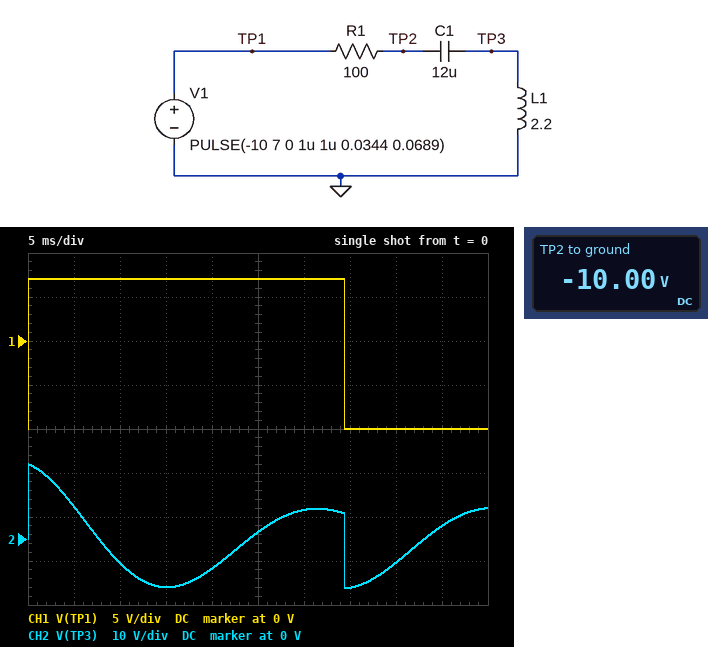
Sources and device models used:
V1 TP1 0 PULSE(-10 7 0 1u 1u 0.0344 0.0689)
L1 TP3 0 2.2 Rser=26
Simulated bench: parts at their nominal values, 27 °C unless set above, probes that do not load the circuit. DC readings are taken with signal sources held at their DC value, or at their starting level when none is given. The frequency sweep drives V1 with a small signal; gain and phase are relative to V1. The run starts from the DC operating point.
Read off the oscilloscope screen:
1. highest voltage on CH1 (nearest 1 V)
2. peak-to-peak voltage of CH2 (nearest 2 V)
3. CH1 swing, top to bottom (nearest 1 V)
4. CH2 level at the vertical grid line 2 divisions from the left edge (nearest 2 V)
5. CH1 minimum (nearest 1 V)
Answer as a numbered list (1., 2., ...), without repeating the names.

1. 7 V
2. 28 V
3. 17 V
4. -6 V
5. -10 V
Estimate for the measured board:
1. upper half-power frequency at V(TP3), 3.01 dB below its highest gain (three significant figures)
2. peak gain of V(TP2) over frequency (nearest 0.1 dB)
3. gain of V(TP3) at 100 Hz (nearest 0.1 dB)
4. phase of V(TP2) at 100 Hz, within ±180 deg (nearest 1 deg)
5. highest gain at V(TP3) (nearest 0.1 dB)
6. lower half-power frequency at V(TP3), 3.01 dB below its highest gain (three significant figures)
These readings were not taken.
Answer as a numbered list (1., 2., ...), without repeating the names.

1. 38.0 Hz
2. 0 dB
3. 0.8 dB
4. 5 deg
5. 10.7 dB
6. 27.7 Hz
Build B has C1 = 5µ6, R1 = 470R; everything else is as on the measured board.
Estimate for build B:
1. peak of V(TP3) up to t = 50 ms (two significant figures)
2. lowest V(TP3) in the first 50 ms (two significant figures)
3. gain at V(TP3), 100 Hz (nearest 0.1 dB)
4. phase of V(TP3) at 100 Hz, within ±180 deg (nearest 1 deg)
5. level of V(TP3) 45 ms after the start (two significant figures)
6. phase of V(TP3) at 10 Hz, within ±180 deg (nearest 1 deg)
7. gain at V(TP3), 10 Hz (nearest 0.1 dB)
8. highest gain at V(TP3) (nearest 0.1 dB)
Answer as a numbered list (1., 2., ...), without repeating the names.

1. 17 V
2. -17 V
3. 1.2 dB
4. 23 deg
5. 5.6 V
6. 159 deg
7. -25.8 dB
8. 2.8 dB
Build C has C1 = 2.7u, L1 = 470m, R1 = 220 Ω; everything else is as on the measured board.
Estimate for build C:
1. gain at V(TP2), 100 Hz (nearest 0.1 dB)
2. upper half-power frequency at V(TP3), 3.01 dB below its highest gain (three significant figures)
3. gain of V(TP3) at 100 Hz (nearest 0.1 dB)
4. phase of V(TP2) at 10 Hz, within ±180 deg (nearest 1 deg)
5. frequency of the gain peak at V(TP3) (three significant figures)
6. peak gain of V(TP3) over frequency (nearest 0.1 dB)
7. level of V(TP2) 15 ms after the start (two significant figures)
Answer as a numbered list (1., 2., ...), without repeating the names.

1. -2.3 dB
2. 275 Hz
3. -2.2 dB
4. -2 deg
5. 155 Hz
6. 5.0 dB
7. 7.0 V
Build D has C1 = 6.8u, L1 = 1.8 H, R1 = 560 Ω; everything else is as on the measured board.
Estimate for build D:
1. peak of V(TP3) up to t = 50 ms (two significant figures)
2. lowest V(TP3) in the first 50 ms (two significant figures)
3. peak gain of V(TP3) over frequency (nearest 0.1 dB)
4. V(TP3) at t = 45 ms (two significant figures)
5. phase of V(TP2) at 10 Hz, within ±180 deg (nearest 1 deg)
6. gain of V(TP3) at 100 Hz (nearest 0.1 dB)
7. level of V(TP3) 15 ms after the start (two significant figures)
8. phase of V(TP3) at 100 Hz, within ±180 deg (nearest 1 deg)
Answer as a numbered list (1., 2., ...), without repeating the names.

1. 17 V
2. -17 V
3. 0.6 dB
4. 3.6 V
5. -14 deg
6. 0.5 dB
7. -1.0 V
8. 32 deg
